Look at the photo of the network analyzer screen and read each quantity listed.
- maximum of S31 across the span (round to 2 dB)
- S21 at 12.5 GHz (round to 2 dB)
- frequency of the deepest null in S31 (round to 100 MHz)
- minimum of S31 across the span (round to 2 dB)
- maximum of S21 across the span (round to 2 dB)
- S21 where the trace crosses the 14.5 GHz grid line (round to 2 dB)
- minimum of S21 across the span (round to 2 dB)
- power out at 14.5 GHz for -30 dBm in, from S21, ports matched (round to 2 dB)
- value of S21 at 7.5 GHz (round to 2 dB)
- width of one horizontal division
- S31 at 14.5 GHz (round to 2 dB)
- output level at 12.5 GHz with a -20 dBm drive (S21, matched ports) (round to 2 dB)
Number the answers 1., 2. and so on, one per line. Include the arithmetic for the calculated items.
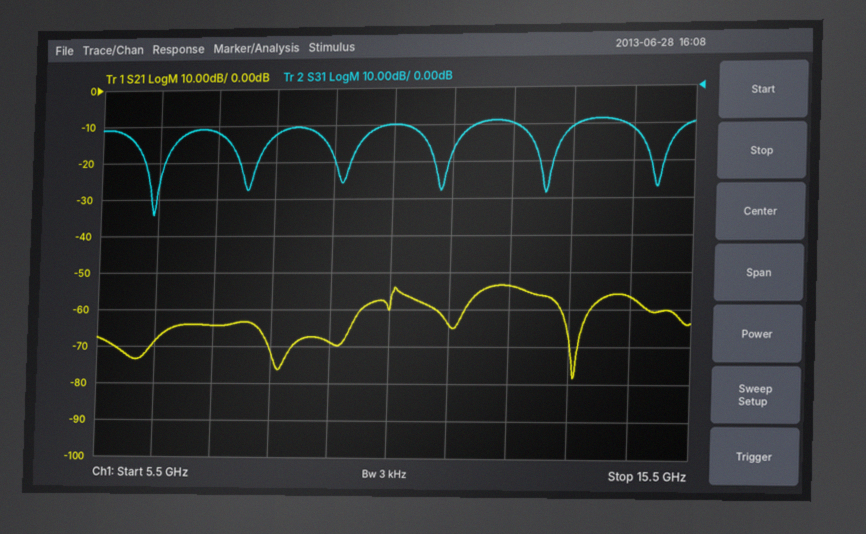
1. -8 dB
2. -54 dB
3. 6.4 GHz
4. -34 dB
5. -54 dB
6. -56 dB
7. -78 dB
8. -30 dBm + (-56 dB) = -86 dBm
9. -64 dB
10. 1 GHz
11. -12 dB
12. -20 dBm + (-54 dB) = -74 dBm
